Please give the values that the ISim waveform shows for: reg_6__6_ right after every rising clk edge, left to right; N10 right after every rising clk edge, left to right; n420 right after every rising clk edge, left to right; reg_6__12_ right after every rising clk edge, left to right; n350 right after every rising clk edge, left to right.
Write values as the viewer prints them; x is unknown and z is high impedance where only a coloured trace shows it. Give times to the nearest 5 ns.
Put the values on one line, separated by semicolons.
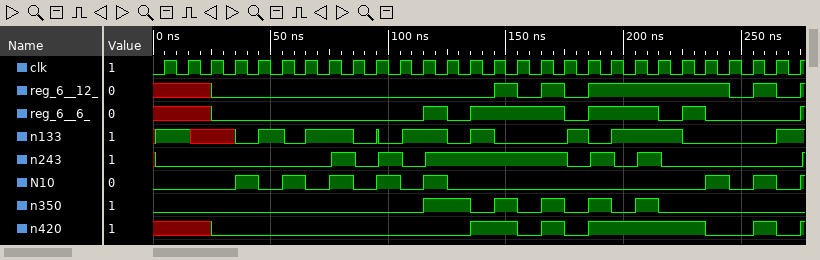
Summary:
x x 0 0 0 0 0 0 0 0 0 1 0 1 1 1 1 0 1 1 1 0 1 0 0 0 0 1; 0 0 0 1 0 1 0 1 0 1 0 1 0 0 0 0 0 0 0 0 0 0 0 1 0 1 0 1; x x 0 0 0 0 0 0 0 0 0 0 0 1 1 0 1 0 1 1 1 1 1 0 0 1 0 1; x x 0 0 0 0 0 0 0 0 0 0 0 0 1 0 1 0 1 1 1 1 1 1 0 1 0 1; 0 0 0 0 0 0 0 0 0 0 0 1 1 0 1 0 1 0 1 0 1 0 0 0 0 0 0 0
